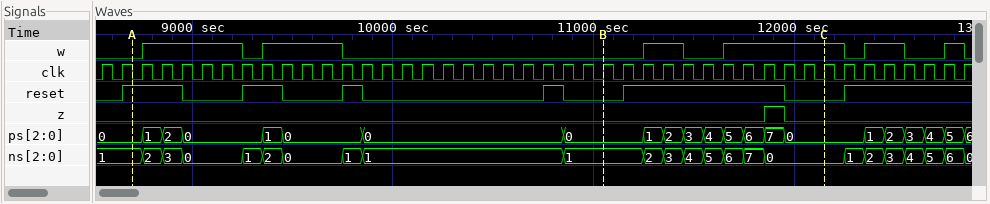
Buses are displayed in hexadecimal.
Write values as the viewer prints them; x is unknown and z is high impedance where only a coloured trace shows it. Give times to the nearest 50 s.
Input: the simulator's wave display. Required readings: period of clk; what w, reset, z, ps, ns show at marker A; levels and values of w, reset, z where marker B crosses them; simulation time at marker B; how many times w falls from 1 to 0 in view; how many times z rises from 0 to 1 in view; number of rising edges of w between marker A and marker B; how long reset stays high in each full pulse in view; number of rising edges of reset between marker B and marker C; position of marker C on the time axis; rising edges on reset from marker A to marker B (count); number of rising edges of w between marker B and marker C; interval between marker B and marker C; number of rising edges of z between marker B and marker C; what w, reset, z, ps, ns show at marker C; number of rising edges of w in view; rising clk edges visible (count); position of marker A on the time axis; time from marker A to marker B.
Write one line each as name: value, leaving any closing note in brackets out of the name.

period of clk: 100 s
what w, reset, z, ps, ns show at marker A: w=0, reset=1, z=0, ps=0, ns=1
levels and values of w, reset, z where marker B crosses them: w=0, reset=0, z=0
simulation time at marker B: 11050 s
how many times w falls from 1 to 0 in view: 6
how many times z rises from 0 to 1 in view: 1
number of rising edges of w between marker A and marker B: 2
how long reset stays high in each full pulse in view: 300 s, 200 s, 100 s, 100 s, 800 s
number of rising edges of reset between marker B and marker C: 1
position of marker C on the time axis: 12150 s
rising edges on reset from marker A to marker B: 3
number of rising edges of w between marker B and marker C: 2
interval between marker B and marker C: 1100 s
number of rising edges of z between marker B and marker C: 1
what w, reset, z, ps, ns show at marker C: w=1, reset=0, z=0, ps=0, ns=0
number of rising edges of w in view: 6
rising clk edges visible: 44
position of marker A on the time axis: 8700 s
time from marker A to marker B: 2350 s
